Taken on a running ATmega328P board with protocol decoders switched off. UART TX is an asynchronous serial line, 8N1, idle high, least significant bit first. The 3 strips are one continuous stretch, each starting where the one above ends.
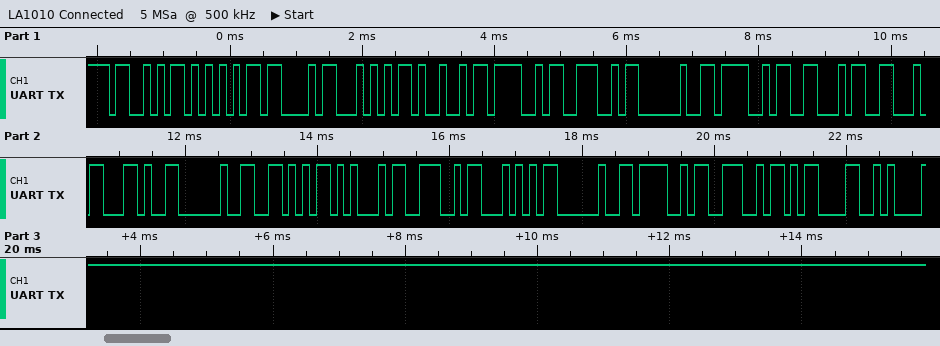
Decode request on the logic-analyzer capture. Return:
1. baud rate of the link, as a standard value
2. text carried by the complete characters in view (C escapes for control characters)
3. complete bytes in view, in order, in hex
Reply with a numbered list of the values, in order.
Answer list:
1. 9600 baud
2. "SUCTION OFF, VENT ON\r\n"
3. 0x53 0x55 0x43 0x54 0x49 0x4F 0x4E 0x20 0x4F 0x46 0x46 0x2C 0x20 0x56 0x45 0x4E 0x54 0x20 0x4F 0x4E 0x0D 0x0A
